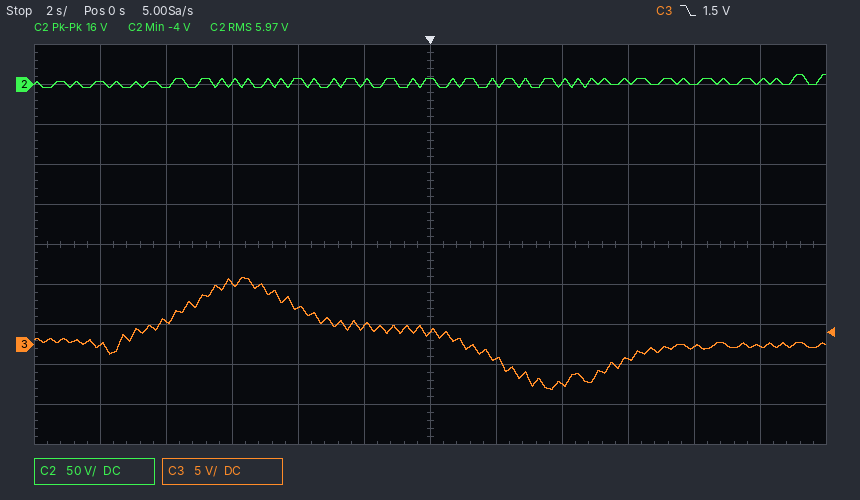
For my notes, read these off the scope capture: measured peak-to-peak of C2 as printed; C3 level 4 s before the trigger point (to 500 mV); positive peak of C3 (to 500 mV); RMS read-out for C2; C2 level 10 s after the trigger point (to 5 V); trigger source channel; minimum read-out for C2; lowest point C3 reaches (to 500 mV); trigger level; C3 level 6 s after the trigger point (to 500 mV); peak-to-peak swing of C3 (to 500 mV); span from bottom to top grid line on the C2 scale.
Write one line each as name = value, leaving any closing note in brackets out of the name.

measured peak-to-peak of C2 as printed = 16 V
C3 level 4 s before the trigger point = 4.5 V
positive peak of C3 = 8.5 V
RMS read-out for C2 = 5.97 V
C2 level 10 s after the trigger point = 5 V
trigger source channel = C3
minimum read-out for C2 = -4 V
lowest point C3 reaches = -5.5 V
trigger level = 1.5 V
C3 level 6 s after the trigger point = -2.0 V
peak-to-peak swing of C3 = 14.0 V
span from bottom to top grid line on the C2 scale = 500 V
